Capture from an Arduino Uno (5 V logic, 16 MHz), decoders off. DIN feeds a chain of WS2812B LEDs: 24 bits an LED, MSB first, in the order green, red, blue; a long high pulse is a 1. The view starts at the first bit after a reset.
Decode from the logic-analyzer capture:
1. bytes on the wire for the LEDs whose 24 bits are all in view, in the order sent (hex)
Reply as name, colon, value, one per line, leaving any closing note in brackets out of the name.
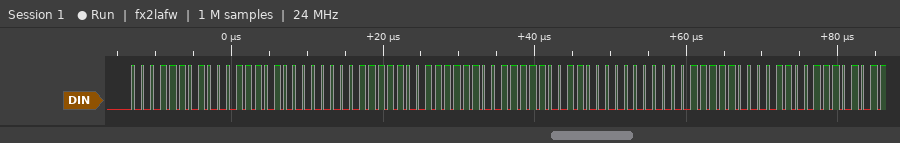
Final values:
bytes on the wire for the LEDs whose 24 bits are all in view, in the order sent: 1D 1D 00 F9 F9 F3 00 1F 0C
